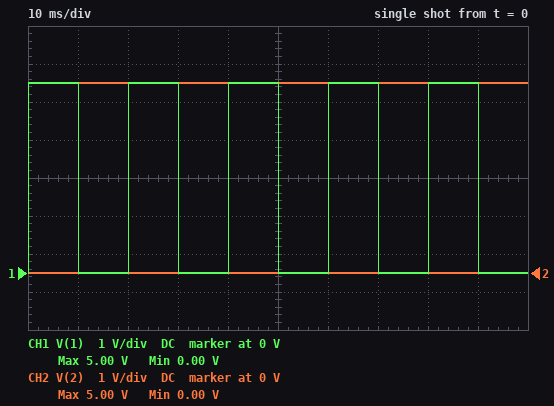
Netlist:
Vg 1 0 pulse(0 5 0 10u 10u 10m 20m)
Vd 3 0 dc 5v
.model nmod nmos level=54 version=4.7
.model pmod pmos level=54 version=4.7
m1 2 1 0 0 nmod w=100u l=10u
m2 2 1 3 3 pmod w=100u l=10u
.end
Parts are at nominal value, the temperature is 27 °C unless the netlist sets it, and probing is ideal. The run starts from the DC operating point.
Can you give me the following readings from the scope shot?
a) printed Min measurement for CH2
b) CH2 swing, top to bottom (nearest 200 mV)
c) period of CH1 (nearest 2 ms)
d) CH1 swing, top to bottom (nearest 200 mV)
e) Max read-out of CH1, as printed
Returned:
0.00 V
5.0 V
20 ms
5.0 V
5.00 V
